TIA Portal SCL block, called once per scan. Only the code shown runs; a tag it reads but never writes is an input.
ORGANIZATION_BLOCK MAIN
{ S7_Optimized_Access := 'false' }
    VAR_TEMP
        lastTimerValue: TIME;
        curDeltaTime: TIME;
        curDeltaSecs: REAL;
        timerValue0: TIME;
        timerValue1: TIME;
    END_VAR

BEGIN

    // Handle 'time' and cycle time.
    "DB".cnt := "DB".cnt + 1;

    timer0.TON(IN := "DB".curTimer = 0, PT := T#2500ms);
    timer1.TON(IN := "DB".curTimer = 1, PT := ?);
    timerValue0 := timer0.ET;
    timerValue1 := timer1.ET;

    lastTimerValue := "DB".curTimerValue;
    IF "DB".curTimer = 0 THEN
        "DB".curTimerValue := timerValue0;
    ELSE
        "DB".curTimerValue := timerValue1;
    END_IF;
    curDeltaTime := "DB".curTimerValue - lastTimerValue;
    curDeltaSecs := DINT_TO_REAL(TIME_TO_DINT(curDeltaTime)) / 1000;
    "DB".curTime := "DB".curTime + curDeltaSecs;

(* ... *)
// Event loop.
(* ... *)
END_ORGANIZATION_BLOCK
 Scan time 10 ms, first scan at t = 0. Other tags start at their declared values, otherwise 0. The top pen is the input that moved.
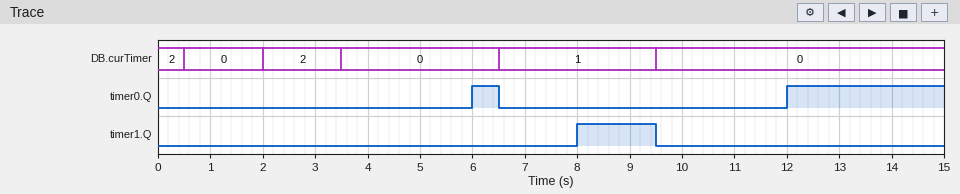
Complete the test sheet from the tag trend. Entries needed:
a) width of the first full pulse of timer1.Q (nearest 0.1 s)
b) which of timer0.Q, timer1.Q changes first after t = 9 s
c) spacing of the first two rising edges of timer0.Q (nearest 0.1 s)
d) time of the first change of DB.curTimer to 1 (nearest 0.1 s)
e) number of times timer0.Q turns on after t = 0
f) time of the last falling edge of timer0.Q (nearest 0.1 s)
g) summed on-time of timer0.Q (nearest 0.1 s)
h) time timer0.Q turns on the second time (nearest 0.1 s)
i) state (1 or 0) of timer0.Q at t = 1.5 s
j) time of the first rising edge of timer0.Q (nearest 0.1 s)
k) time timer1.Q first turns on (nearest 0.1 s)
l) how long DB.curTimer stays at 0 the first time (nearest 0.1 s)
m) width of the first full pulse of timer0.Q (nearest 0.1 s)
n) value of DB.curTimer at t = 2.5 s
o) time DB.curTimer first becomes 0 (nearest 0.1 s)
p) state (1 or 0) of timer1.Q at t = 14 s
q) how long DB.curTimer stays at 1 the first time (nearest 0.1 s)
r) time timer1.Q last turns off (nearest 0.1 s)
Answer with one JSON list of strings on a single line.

["1.5 s", "timer1.Q", "6.0 s", "6.5 s", "2", "6.5 s", "3.5 s", "12.0 s", "0", "6.0 s", "8.0 s", "1.5 s", "0.5 s", "2", "0.5 s", "0", "3.0 s", "9.5 s"]
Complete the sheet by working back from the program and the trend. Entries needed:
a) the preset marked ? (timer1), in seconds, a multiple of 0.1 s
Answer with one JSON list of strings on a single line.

["1.5 s"]
